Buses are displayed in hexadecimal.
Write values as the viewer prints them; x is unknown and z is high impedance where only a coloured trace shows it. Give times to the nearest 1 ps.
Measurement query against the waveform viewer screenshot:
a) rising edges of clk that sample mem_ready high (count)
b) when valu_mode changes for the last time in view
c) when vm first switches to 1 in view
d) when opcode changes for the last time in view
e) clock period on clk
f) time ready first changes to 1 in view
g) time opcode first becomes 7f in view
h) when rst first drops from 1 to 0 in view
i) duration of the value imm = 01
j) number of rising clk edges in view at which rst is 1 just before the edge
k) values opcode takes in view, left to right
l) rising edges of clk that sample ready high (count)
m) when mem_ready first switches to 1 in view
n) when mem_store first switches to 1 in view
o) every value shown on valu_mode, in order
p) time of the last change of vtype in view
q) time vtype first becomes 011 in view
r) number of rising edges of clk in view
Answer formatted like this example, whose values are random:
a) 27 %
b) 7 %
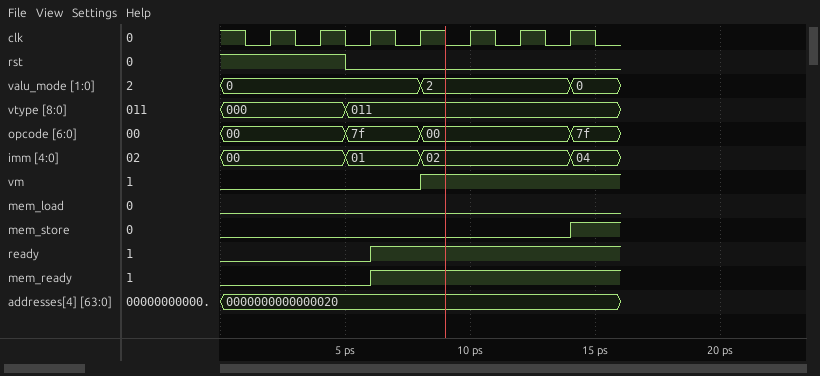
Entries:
a) 4
b) 14 ps
c) 8 ps
d) 14 ps
e) 2 ps
f) 6 ps
g) 5 ps
h) 5 ps
i) 3 ps
j) 2
k) 00, 7f, 00, 7f
l) 4
m) 6 ps
n) 14 ps
o) 0, 2, 0
p) 5 ps
q) 5 ps
r) 7
